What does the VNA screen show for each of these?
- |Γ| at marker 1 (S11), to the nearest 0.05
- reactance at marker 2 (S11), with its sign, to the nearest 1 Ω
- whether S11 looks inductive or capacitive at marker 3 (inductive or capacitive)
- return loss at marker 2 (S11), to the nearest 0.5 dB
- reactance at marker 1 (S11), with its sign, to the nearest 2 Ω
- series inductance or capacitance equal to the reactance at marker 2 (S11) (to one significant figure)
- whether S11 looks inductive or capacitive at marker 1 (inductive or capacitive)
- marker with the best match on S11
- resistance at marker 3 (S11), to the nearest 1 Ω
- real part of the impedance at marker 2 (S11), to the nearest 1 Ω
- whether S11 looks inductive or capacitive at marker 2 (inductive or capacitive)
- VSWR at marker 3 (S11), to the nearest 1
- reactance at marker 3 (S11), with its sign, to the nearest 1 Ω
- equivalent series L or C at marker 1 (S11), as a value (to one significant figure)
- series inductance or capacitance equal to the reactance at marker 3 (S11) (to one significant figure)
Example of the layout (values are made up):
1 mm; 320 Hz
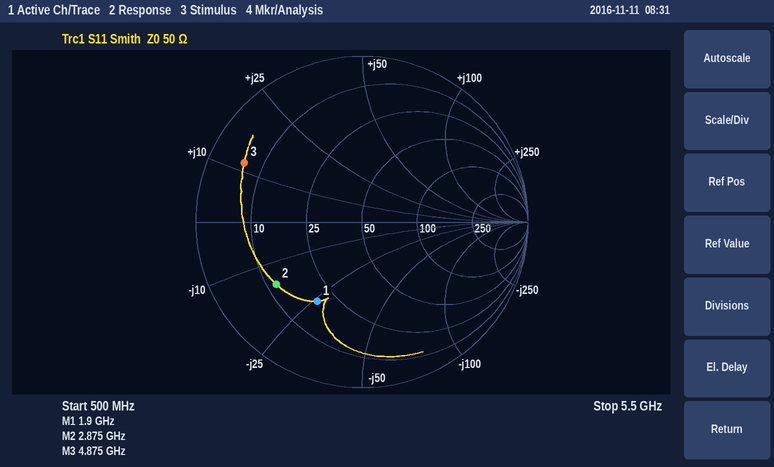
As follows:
0.55; -15 Ω; inductive; 4.0 dB; -26 Ω; 4 pF; capacitive; marker 1; 6 Ω; 12 Ω; capacitive; 9; +12 Ω; 3 pF; 400 pH
